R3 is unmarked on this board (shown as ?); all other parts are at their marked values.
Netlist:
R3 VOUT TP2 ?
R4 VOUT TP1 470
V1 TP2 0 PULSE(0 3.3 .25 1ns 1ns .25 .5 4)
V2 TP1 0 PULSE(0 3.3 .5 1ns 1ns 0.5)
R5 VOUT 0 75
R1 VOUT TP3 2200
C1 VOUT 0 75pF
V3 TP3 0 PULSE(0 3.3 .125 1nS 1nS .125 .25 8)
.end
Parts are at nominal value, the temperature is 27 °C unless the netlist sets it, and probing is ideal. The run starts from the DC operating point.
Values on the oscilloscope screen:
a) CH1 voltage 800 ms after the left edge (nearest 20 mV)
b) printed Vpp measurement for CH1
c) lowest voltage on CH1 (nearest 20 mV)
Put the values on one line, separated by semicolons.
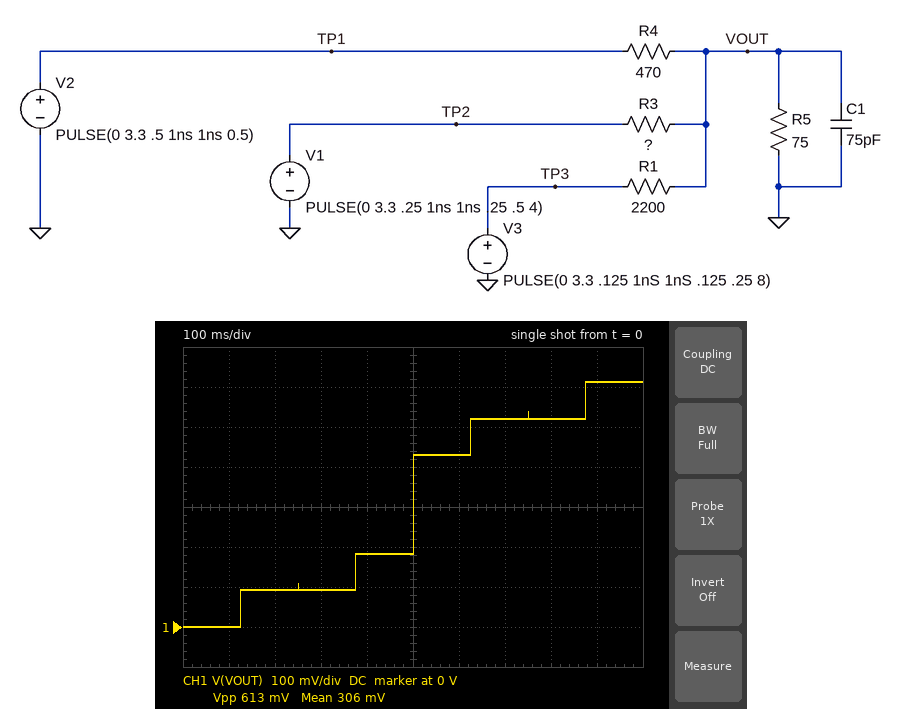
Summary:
520 mV; 613 mV; 0 V
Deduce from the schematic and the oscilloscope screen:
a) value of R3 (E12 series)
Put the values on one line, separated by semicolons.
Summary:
2.2 kΩ
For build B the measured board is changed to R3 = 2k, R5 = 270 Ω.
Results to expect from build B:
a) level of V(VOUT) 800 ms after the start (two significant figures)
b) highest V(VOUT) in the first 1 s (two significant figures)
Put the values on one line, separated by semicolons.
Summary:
1.3 V; 1.5 V
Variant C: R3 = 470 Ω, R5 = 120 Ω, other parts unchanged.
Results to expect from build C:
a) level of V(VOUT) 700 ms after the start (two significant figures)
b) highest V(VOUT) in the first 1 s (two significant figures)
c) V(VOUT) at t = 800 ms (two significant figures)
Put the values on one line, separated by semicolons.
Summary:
650 mV; 1.2 V; 1.1 V
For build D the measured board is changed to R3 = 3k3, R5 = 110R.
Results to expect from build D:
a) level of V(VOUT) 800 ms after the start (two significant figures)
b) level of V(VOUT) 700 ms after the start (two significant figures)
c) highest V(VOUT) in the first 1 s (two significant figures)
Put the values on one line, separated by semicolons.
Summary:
670 mV; 710 mV; 800 mV
